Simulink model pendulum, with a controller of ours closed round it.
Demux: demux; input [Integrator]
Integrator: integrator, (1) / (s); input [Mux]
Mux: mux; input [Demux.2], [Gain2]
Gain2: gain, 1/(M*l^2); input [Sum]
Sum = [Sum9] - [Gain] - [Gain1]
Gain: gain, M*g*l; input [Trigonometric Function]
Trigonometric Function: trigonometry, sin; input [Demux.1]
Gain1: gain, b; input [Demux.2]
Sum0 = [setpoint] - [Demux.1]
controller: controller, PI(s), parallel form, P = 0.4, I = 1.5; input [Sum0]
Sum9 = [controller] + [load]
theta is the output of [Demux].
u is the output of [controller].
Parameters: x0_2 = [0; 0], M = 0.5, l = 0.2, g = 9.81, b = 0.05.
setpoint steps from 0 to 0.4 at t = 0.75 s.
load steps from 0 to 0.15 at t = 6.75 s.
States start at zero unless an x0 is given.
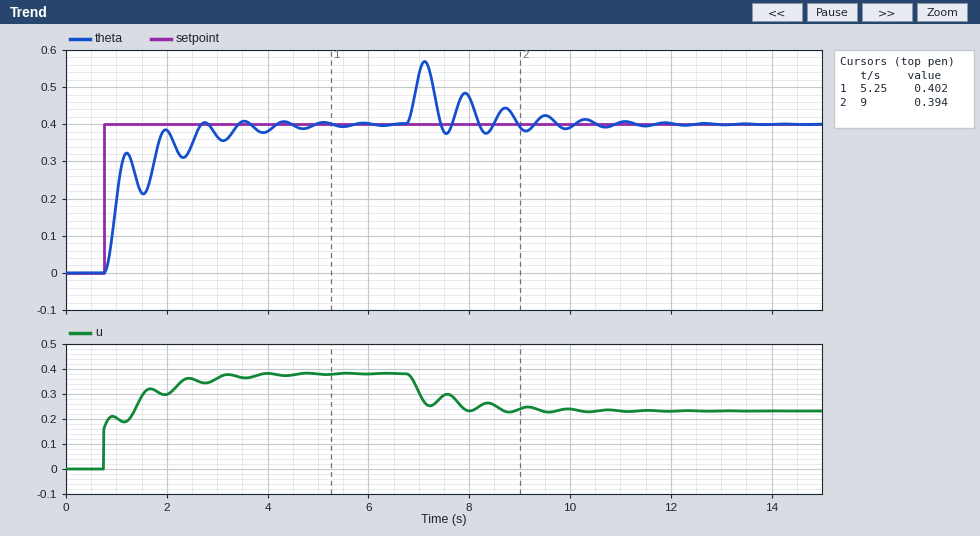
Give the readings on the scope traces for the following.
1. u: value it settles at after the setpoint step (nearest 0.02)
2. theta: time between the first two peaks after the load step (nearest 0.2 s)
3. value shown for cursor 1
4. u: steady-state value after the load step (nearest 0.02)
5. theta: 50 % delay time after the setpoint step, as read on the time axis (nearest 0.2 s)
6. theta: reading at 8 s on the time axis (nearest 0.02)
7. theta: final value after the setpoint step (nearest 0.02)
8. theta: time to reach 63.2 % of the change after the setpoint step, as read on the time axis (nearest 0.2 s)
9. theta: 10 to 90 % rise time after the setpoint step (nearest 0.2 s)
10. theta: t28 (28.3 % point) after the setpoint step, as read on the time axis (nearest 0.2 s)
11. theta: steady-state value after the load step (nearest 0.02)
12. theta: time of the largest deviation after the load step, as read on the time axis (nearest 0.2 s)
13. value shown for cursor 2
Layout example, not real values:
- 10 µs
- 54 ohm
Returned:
- 0.38
- 0.8 s
- 0.402
- 0.24
- 1.0 s
- 0.48
- 0.40
- 1.0 s
- 1.0 s
- 1.0 s
- 0.40
- 7.2 s
- 0.394
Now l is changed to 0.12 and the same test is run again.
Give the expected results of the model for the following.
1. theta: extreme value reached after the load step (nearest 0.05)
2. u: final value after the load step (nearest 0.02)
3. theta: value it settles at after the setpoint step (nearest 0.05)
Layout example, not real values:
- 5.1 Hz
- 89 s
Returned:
- 0.60
- 0.08
- 0.40
